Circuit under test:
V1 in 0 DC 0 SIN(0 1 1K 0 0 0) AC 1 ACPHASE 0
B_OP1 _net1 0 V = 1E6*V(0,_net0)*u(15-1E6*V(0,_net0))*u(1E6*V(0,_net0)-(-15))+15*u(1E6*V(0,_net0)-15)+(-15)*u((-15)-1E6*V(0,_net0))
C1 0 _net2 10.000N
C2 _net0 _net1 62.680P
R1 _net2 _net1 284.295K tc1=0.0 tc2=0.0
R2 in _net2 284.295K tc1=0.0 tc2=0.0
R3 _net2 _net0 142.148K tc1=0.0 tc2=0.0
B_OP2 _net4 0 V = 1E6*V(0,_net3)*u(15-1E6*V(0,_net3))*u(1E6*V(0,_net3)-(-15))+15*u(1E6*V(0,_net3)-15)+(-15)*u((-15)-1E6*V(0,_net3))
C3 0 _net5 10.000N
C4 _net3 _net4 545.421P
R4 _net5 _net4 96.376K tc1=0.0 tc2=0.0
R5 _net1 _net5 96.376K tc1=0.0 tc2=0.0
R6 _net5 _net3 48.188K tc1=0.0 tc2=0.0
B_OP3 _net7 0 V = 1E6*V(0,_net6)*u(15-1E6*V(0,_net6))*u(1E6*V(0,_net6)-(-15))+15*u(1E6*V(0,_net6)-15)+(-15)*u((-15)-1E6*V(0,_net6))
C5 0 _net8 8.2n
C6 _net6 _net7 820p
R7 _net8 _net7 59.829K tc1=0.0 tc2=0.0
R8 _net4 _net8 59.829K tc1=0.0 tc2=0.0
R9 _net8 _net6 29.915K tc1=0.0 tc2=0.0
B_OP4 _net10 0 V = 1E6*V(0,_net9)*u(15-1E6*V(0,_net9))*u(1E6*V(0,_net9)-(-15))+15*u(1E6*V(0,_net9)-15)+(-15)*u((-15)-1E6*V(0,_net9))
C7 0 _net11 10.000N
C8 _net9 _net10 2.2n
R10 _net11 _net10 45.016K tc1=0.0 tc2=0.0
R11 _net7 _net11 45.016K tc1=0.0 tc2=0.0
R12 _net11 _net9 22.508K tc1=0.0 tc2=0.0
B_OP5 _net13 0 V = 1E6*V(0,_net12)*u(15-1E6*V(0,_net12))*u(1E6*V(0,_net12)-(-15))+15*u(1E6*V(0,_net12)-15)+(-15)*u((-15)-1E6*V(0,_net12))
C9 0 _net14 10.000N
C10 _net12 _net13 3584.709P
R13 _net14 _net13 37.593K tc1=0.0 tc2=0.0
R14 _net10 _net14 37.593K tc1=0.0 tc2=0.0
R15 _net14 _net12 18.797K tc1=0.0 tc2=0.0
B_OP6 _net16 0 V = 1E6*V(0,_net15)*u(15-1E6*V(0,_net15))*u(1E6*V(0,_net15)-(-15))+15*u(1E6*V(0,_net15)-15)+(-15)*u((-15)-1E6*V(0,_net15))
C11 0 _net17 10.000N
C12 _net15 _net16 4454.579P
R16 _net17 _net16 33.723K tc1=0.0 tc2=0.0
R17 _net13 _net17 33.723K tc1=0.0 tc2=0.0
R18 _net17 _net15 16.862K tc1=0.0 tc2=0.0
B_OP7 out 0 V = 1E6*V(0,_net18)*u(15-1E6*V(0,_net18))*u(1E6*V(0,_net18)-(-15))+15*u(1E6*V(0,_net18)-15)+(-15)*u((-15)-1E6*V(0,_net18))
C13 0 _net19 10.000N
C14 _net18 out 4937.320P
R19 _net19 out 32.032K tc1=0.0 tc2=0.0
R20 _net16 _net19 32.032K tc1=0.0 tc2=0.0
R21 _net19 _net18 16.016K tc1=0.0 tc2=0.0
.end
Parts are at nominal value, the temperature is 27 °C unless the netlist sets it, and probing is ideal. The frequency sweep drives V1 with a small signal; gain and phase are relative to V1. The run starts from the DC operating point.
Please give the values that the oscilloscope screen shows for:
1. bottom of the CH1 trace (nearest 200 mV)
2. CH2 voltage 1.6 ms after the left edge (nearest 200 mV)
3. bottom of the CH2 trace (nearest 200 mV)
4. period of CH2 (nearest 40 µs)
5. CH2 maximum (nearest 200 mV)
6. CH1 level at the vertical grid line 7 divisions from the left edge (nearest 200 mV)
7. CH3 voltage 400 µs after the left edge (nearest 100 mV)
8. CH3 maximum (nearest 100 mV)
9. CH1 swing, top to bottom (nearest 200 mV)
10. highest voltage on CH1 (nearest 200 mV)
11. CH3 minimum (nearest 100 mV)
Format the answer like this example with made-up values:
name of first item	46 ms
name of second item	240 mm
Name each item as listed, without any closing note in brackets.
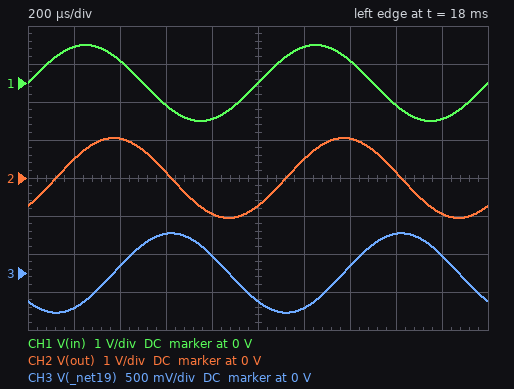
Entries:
bottom of the CH1 trace	-1.0 V
CH2 voltage 1.6 ms after the left edge	200 mV
bottom of the CH2 trace	-1.0 V
period of CH2	1.00 ms
CH2 maximum	1.0 V
CH1 level at the vertical grid line 7 divisions from the left edge	600 mV
CH3 voltage 400 µs after the left edge	100 mV
CH3 maximum	500 mV
CH1 swing, top to bottom	2.0 V
highest voltage on CH1	1.0 V
CH3 minimum	-500 mV
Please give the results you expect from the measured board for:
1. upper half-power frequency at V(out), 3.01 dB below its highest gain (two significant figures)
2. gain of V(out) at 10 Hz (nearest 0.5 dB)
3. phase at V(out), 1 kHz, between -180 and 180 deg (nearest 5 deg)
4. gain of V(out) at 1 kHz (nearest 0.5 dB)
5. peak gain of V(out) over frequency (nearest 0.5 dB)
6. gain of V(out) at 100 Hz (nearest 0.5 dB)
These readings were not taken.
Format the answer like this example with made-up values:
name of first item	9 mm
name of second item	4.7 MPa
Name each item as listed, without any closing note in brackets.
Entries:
upper half-power frequency at V(out), 3.01 dB below its highest gain	1.0 kHz
gain of V(out) at 10 Hz	0 dB
phase at V(out), 1 kHz, between -180 and 180 deg	-45 deg
gain of V(out) at 1 kHz	0.5 dB
peak gain of V(out) over frequency	2.0 dB
gain of V(out) at 100 Hz	0 dB
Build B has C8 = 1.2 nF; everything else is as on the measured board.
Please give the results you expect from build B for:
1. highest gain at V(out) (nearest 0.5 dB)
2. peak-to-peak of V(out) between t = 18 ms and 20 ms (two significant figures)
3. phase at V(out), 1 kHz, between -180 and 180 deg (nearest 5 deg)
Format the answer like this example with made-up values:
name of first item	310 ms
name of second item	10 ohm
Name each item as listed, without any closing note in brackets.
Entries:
highest gain at V(out)	5.0 dB
peak-to-peak of V(out) between t = 18 ms and 20 ms	3.1 V
phase at V(out), 1 kHz, between -180 and 180 deg	-10 deg
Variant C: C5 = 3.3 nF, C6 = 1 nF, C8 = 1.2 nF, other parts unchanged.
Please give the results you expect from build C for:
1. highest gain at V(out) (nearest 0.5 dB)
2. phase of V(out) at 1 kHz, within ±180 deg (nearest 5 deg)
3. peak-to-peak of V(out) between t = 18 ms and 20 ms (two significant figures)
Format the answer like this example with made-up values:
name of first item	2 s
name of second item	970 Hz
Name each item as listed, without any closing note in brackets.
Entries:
highest gain at V(out)	2.5 dB
phase of V(out) at 1 kHz, within ±180 deg	-5 deg
peak-to-peak of V(out) between t = 18 ms and 20 ms	2.3 V
